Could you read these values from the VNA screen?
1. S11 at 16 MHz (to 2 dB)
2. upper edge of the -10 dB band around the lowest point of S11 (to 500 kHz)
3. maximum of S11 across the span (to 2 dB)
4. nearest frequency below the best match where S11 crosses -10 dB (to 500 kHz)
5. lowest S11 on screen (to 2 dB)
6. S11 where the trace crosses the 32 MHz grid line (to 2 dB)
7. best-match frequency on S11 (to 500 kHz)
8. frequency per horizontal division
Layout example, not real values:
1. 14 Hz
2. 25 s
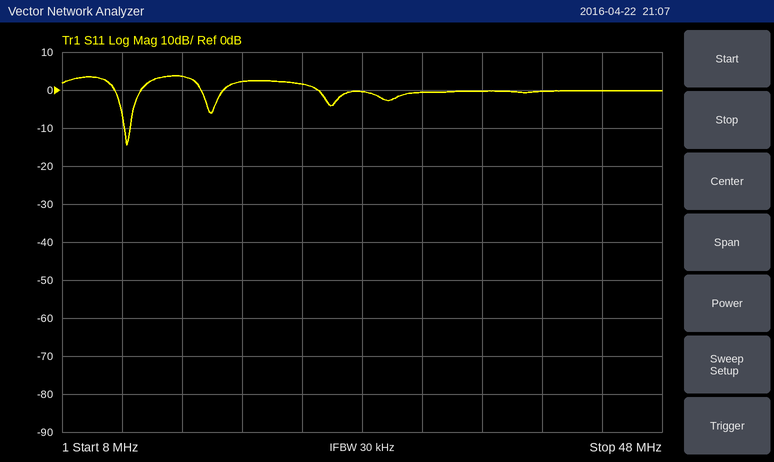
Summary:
1. 4 dB
2. 12.5 MHz
3. 4 dB
4. 12.0 MHz
5. -14 dB
6. 0 dB
7. 12.5 MHz
8. 4 MHz
